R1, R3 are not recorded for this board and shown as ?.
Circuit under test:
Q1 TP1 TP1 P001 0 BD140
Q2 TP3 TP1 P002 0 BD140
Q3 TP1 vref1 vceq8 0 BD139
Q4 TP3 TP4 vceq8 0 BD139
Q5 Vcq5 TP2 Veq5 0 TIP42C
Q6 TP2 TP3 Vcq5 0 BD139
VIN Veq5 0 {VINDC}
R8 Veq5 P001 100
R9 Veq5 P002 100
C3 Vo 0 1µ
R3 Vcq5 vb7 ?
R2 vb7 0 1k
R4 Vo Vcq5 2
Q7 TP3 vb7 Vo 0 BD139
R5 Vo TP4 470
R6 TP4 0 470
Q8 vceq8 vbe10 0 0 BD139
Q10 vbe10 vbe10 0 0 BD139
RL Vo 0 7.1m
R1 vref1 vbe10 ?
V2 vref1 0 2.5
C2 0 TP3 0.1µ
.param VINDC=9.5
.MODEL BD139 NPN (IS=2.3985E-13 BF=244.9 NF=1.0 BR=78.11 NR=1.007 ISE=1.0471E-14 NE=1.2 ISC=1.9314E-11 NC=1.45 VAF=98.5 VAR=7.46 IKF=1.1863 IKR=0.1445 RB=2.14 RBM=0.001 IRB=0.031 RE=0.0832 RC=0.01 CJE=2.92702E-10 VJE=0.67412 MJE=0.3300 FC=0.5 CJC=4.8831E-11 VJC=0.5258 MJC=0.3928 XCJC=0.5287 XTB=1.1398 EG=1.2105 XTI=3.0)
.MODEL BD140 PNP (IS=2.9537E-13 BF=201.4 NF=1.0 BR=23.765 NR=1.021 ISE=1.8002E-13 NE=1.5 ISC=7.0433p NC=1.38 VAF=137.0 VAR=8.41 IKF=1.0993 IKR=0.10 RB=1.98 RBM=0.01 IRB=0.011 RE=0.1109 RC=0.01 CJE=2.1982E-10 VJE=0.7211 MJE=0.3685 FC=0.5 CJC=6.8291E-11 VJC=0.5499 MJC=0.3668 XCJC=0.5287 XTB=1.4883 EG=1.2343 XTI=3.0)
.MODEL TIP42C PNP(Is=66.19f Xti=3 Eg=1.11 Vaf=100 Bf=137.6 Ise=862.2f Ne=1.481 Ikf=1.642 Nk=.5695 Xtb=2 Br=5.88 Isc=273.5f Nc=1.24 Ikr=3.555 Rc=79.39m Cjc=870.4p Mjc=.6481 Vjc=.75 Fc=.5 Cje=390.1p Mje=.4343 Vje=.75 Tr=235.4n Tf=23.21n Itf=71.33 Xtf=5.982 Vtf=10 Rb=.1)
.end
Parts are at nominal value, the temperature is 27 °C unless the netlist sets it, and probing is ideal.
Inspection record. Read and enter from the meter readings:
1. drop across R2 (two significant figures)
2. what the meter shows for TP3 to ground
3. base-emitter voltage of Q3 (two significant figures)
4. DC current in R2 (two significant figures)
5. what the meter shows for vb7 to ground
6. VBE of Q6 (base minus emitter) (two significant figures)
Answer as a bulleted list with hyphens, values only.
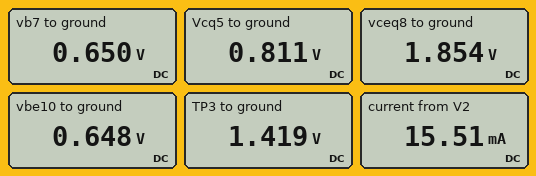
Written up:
- 650 mV
- 1.419 V
- 650 mV
- 650 µA
- 0.650 V
- 610 mV
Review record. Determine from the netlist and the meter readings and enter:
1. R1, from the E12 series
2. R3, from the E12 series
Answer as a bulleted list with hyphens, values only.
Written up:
- 120 Ω
- 220 Ω
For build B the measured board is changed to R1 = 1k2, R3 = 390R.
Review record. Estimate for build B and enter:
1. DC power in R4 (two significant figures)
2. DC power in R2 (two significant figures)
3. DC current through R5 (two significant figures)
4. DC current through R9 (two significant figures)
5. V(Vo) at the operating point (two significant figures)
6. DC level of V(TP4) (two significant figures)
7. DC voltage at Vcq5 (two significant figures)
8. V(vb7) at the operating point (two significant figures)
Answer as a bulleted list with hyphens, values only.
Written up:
- 340 mW
- 350 µW
- 3.1 µA
- 1.6 mA
- 2.9 mV
- 1.5 mV
- 820 mV
- 590 mV
